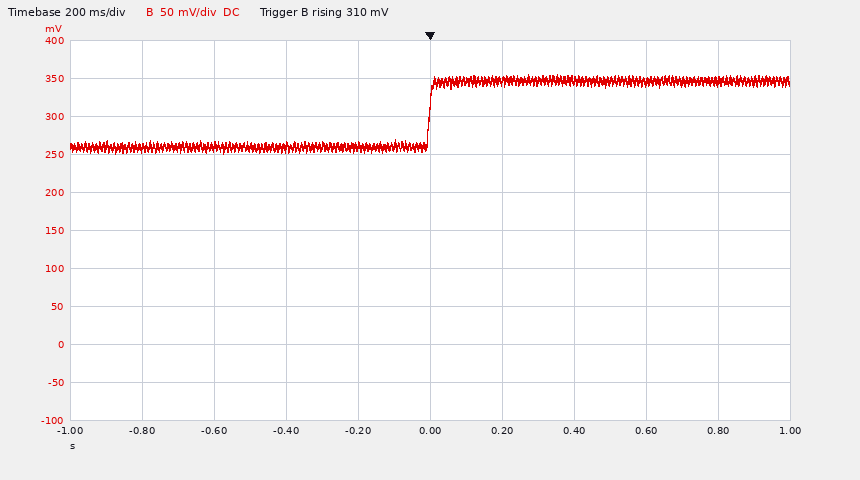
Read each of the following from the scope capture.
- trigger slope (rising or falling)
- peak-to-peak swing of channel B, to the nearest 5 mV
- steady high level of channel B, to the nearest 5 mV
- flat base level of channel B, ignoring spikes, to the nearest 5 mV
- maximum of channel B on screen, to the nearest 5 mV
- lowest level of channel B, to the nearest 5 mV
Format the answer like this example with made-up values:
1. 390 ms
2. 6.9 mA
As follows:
1. rising
2. 105 mV
3. 345 mV
4. 260 mV
5. 355 mV
6. 250 mV
